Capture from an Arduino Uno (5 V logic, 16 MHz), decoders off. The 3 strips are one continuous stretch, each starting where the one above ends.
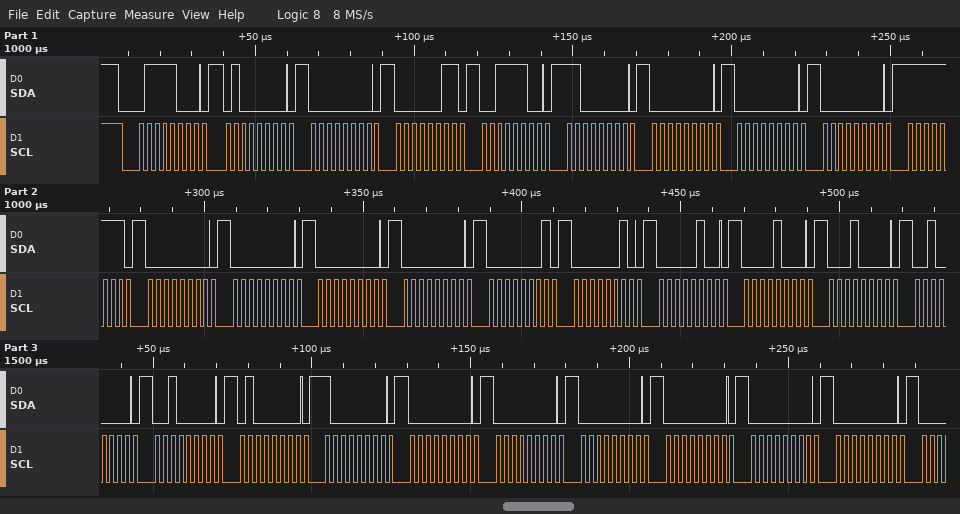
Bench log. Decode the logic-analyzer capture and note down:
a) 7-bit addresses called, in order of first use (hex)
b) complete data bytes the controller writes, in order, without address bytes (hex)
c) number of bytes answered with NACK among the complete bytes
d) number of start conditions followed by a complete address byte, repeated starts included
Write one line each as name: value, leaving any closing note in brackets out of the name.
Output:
7-bit addresses called, in order of first use: 0x3C
complete data bytes the controller writes, in order, without address bytes: 40 00 03 3C C0 00 00 00 FF 00 00 00 00 01 02 04 08 10 20 20 40 80 00 00 00 00 00 00
number of bytes answered with NACK among the complete bytes: 0
number of start conditions followed by a complete address byte, repeated starts included: 1
